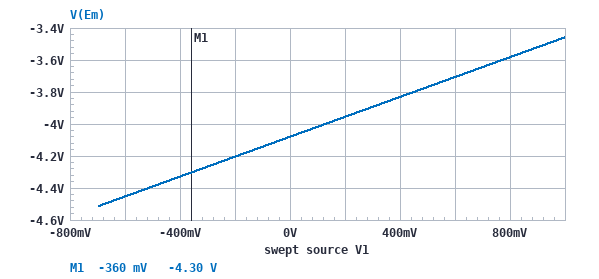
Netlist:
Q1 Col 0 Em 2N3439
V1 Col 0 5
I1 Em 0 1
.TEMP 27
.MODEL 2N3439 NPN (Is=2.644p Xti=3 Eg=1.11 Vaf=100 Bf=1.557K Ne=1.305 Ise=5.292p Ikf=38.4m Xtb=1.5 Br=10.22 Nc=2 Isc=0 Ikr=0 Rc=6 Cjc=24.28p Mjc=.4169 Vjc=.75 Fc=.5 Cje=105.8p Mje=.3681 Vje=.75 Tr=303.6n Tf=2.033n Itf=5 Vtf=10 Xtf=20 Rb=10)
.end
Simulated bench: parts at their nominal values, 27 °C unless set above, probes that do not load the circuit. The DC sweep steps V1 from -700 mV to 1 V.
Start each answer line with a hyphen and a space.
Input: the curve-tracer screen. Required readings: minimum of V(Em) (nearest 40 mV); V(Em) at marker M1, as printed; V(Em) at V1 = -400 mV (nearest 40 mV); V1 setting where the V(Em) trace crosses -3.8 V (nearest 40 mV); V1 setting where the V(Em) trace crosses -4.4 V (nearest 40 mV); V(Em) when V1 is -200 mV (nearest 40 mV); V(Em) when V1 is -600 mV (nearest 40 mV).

- -4.52 V
- -4.30 V
- -4.32 V
- 440 mV
- -520 mV
- -4.20 V
- -4.44 V
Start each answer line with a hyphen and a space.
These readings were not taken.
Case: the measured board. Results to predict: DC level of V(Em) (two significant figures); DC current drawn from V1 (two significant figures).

- -1.4 V
- 940 mA
